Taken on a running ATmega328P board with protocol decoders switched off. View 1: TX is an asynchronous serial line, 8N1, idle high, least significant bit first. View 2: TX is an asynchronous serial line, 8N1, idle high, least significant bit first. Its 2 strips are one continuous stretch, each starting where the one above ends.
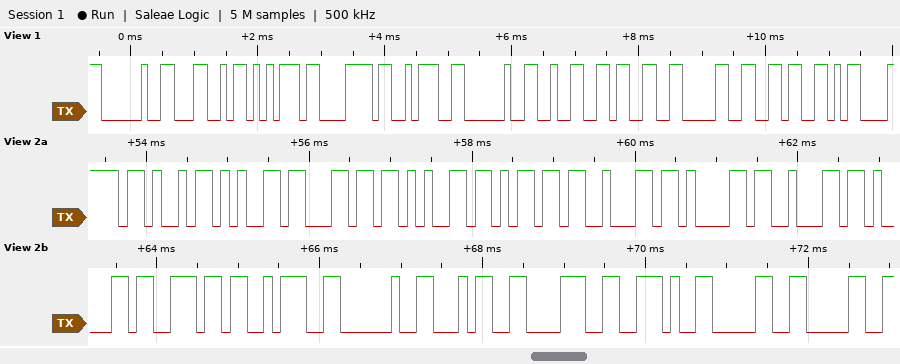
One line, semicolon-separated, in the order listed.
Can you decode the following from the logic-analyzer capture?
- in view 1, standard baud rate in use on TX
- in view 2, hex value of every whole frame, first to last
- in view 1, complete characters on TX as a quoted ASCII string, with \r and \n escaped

9600 baud; 4B 65 6C 65 6D 62 61 62 61 6E 3A 20 34 38 2E 30 30; " Lux: 2306\r"
